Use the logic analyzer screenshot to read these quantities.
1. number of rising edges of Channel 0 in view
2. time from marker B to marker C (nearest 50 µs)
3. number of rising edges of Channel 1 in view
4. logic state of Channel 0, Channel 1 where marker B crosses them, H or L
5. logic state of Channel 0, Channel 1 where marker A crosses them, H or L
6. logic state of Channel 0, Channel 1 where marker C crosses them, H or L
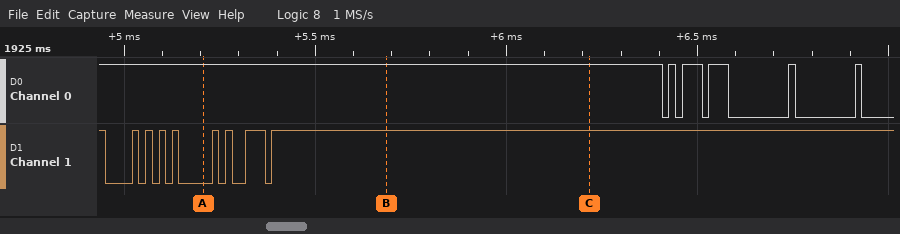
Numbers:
5
550 µs
8
Channel 0=H, Channel 1=H
Channel 0=H, Channel 1=L
Channel 0=H, Channel 1=H
